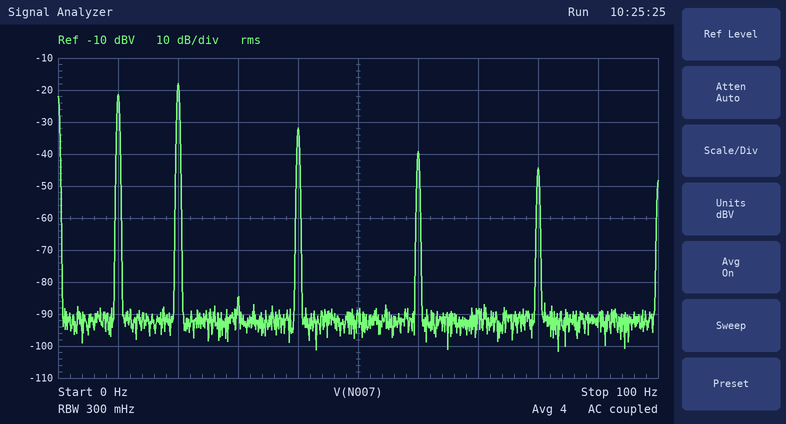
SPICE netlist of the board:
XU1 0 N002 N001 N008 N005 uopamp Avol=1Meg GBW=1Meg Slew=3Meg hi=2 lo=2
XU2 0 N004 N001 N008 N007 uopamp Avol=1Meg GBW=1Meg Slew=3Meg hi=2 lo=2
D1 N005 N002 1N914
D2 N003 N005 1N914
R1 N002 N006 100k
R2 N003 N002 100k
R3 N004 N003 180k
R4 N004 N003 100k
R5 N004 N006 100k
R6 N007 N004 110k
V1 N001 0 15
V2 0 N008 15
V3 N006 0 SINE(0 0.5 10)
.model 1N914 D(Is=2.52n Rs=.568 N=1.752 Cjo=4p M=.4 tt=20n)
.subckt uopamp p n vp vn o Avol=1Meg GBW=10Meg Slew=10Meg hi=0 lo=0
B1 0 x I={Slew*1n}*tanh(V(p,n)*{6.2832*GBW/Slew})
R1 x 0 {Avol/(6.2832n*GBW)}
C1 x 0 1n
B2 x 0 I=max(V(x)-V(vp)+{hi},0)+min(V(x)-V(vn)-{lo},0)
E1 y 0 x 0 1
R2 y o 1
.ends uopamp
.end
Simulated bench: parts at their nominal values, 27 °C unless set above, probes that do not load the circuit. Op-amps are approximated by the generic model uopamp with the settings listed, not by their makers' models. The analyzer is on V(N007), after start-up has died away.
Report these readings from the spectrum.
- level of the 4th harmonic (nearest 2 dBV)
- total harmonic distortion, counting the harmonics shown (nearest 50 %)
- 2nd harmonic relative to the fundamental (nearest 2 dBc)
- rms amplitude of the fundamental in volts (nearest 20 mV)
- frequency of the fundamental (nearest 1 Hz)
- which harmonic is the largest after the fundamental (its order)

-32 dBV
150 %
4 dBc
80 mV
10 Hz
2
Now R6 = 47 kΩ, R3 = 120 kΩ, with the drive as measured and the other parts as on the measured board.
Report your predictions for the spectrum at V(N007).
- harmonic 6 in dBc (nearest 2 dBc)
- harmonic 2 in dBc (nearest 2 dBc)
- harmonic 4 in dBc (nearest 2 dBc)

-8 dBc
14 dBc
0 dBc
